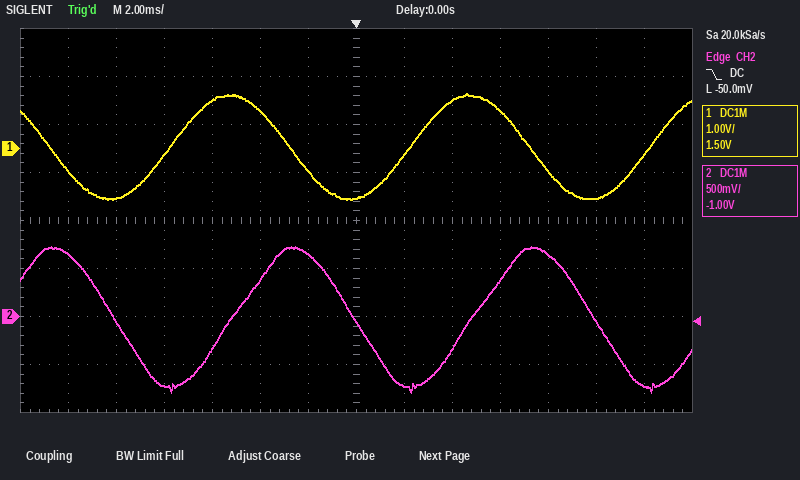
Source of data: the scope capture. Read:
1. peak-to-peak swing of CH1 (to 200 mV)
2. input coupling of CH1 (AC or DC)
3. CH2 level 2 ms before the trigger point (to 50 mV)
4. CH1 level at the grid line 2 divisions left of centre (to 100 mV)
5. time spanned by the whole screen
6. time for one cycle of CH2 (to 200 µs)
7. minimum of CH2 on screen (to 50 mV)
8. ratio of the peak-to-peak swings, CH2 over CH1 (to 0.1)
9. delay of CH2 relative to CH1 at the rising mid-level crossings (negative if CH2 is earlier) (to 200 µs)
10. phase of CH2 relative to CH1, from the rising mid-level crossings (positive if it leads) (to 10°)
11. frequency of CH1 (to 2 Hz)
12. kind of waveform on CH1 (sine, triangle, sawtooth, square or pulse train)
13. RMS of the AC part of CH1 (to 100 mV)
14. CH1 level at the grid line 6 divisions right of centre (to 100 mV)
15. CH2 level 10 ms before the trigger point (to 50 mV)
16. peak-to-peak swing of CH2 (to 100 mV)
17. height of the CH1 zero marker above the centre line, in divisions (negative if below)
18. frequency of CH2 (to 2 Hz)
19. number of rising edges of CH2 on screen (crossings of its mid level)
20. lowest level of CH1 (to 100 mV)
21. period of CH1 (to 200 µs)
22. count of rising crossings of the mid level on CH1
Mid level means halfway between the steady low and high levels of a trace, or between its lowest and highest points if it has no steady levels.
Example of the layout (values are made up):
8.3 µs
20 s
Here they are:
2.2 V
DC
650 mV
800 mV
28 ms
10.0 ms
-800 mV
0.7
+2.4 ms
-90°
100 Hz
sine
800 mV
-100 mV
-50 mV
1.50 V
+1.5 div
100 Hz
2
-1.1 V
10.0 ms
3
